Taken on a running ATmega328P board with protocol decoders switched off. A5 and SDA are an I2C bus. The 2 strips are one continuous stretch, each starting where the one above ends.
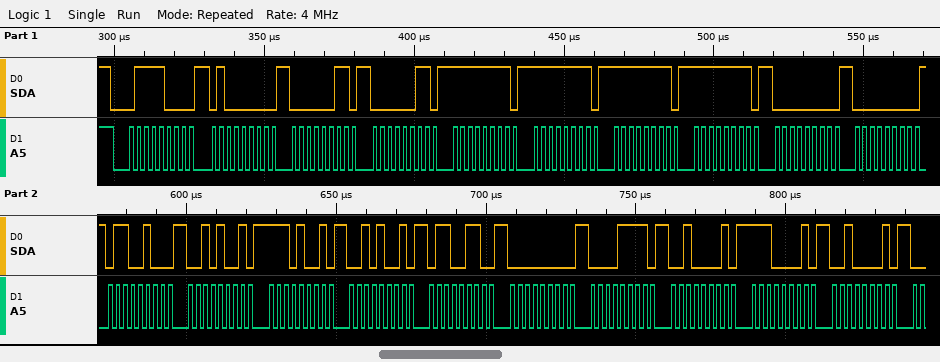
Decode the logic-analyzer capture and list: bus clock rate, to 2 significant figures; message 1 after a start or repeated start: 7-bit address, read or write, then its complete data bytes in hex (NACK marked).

400 kHz
0x3C write: 40 03 03 FF FF FF FF 00 00 64 29 E9 29 66 00 0F 21 E1 21
